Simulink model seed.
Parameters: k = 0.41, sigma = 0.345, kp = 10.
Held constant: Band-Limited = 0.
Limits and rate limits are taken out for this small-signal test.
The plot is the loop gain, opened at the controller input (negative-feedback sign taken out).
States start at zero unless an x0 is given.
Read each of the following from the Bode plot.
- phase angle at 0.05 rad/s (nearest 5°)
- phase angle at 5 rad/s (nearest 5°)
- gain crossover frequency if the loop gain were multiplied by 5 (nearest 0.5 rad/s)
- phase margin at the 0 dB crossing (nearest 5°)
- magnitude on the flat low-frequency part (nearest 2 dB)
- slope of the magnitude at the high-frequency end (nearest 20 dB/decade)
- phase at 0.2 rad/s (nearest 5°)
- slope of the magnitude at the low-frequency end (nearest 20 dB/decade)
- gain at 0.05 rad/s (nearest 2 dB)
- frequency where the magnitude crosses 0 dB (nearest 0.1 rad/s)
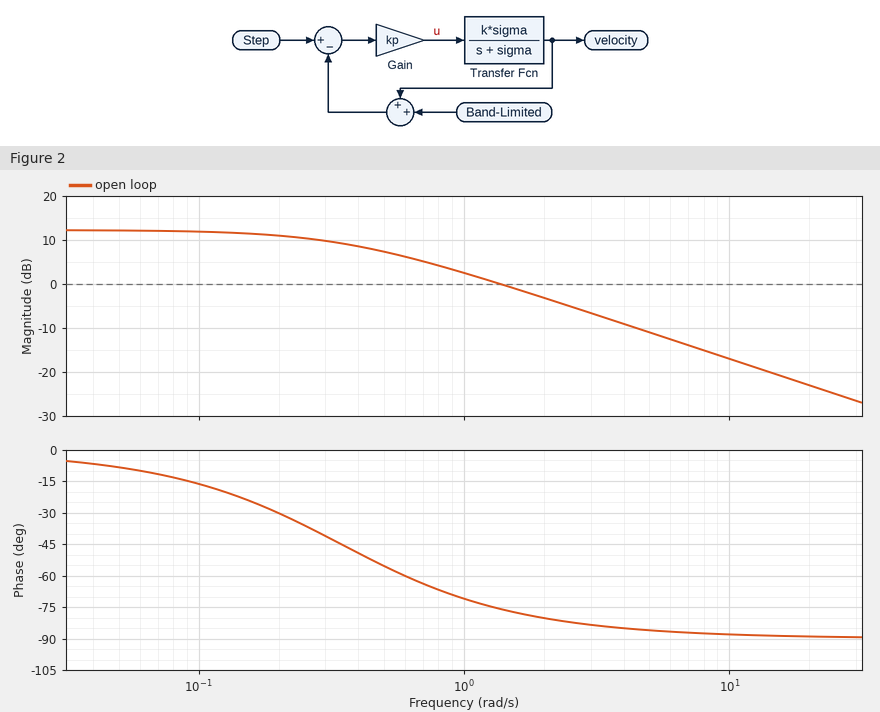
-10°
-85°
7.0 rad/s
105°
12 dB
-20 dB/decade
-30°
0 dB/decade
12 dB
1.4 rad/s
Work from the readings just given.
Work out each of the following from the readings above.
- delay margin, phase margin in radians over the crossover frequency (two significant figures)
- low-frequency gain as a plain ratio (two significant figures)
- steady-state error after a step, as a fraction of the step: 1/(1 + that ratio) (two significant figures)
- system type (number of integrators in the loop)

1.3 s
4.0
0.20
0
